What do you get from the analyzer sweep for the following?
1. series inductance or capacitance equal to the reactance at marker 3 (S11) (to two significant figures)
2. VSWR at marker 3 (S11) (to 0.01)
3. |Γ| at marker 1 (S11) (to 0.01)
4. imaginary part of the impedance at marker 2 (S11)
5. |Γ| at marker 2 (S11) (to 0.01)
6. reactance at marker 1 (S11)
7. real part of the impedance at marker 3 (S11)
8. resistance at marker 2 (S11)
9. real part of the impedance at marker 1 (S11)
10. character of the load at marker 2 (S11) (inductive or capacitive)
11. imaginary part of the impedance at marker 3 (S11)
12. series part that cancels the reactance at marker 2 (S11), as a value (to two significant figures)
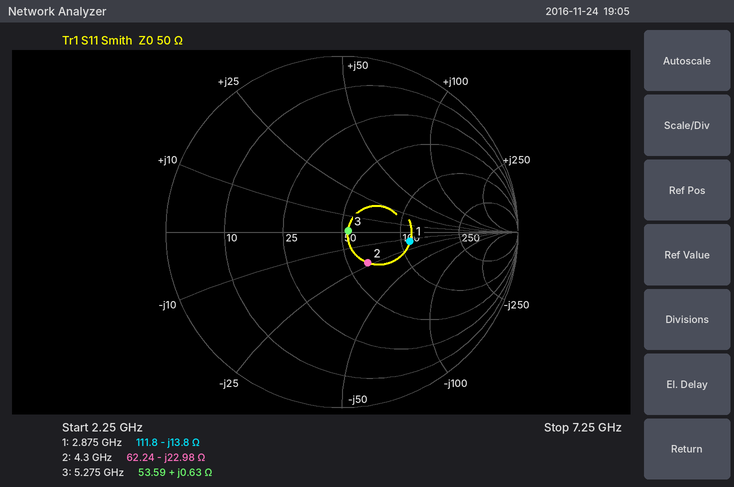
19 pH
1.07
0.39
-22.98 Ω
0.23
-13.8 Ω
53.59 Ω
62.24 Ω
111.8 Ω
capacitive
+0.63 Ω
850 pH
